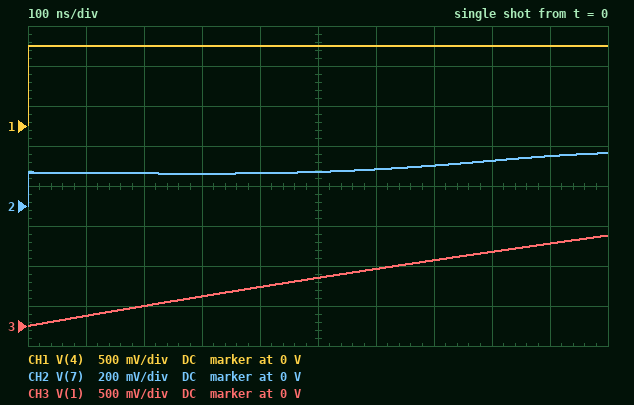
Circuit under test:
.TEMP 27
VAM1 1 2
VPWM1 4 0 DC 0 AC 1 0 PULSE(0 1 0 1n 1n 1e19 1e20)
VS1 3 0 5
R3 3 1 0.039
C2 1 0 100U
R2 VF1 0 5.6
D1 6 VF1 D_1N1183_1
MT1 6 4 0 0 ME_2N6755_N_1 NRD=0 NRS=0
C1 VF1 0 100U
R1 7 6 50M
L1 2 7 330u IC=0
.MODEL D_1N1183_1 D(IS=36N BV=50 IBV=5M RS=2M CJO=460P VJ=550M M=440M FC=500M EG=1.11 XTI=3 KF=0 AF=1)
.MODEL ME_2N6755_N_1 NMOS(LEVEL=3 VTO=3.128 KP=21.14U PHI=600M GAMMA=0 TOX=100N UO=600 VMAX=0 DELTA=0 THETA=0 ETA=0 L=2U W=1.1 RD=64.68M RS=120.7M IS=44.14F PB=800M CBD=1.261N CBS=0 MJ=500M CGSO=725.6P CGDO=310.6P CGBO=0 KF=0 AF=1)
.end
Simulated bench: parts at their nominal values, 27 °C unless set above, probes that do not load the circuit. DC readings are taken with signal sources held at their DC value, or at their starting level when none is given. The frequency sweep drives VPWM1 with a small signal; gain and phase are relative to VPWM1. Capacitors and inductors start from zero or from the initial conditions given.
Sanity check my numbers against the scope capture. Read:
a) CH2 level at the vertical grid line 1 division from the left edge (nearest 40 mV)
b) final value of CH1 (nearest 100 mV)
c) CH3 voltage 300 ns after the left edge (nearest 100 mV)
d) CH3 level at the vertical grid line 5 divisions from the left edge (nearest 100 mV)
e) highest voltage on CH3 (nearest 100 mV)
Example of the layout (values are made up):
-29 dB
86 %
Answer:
160 mV
1.0 V
400 mV
600 mV
1.1 V
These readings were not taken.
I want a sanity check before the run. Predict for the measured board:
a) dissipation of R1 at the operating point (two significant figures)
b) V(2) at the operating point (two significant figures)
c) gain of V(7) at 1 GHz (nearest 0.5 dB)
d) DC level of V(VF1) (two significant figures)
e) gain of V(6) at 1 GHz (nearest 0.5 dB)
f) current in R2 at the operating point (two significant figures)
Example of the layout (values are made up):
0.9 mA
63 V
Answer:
32 mW
5.0 V
-24.0 dB
4.5 V
-24.0 dB
800 mA
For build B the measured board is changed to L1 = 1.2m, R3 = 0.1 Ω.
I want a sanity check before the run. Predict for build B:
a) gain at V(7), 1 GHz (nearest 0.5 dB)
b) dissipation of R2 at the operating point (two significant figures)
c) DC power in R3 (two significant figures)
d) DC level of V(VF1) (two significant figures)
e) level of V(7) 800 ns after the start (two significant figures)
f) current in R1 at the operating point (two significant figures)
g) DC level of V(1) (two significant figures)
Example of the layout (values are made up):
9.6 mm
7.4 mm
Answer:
-24.0 dB
3.5 W
63 mW
4.4 V
160 mV
790 mA
4.9 V
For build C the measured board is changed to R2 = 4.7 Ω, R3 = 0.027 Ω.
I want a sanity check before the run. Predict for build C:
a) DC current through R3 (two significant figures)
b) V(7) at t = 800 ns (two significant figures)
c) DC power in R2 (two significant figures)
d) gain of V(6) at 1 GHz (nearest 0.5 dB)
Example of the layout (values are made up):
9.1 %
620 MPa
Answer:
950 mA
260 mV
4.3 W
-25.0 dB
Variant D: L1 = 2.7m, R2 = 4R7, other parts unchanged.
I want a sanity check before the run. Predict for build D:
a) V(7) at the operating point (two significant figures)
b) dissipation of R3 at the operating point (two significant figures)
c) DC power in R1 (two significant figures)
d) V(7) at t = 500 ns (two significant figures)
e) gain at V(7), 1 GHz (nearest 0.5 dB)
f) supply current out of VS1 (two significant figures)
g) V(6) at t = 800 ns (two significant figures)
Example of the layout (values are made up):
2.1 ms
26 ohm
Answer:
5.0 V
35 mW
45 mW
160 mV
-25.0 dB
950 mA
170 mV
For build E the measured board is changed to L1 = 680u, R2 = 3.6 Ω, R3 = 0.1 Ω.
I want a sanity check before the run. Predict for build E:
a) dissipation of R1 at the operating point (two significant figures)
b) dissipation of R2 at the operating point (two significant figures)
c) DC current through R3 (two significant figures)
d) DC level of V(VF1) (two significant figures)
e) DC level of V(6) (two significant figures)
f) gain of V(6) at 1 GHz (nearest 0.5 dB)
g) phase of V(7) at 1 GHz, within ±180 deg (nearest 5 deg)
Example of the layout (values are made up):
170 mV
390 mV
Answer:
74 mW
5.3 W
1.2 A
4.4 V
4.8 V
-27.0 dB
60 deg
